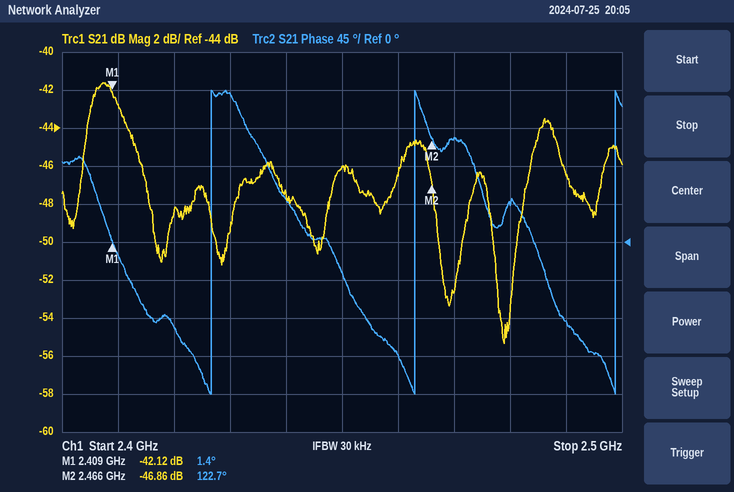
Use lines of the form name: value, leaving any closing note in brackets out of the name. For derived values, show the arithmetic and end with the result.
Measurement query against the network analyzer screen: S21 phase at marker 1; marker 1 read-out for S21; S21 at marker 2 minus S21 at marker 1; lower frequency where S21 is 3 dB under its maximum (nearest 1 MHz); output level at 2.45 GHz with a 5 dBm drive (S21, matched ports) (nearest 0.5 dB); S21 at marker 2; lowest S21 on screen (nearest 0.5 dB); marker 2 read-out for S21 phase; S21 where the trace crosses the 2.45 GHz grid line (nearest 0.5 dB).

S21 phase at marker 1: 1.4°
marker 1 read-out for S21: -42.12 dB
S21 at marker 2 minus S21 at marker 1: -46.86 − (-42.12) = -4.74 dB
lower frequency where S21 is 3 dB under its maximum: 2.404 GHz
output level at 2.45 GHz with a 5 dBm drive (S21, matched ports): 5 dBm + (-46.0 dB) = -41.0 dBm
S21 at marker 2: -46.86 dB
lowest S21 on screen: -55.5 dB
marker 2 read-out for S21 phase: 122.7°
S21 where the trace crosses the 2.45 GHz grid line: -46.0 dB
